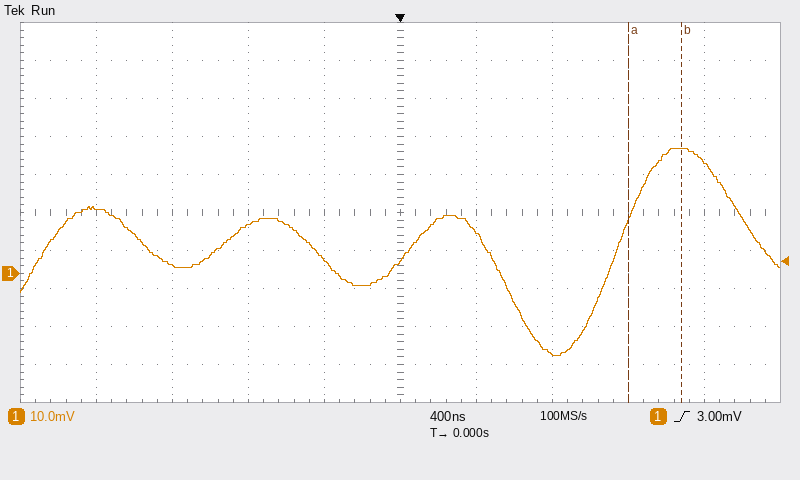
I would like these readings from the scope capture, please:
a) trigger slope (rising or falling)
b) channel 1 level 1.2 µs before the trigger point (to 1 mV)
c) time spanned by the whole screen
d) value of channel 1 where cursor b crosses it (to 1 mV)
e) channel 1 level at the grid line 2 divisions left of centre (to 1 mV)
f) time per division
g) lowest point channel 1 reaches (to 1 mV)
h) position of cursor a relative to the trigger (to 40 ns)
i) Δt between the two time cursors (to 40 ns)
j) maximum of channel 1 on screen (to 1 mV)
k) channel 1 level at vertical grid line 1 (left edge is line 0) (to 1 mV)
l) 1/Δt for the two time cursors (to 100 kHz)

rising
2 mV
4 µs
33 mV
13 mV
400 ns
-22 mV
+1.20 µs
280 ns
33 mV
17 mV
3.6 MHz
